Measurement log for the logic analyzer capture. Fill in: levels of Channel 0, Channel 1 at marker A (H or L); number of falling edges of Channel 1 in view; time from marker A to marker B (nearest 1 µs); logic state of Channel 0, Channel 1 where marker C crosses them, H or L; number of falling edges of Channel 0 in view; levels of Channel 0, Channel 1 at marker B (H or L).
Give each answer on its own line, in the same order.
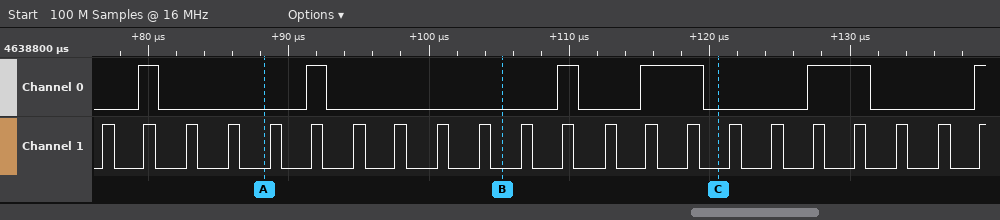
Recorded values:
Channel 0=L, Channel 1=L
21
17 µs
Channel 0=L, Channel 1=L
5
Channel 0=L, Channel 1=L
